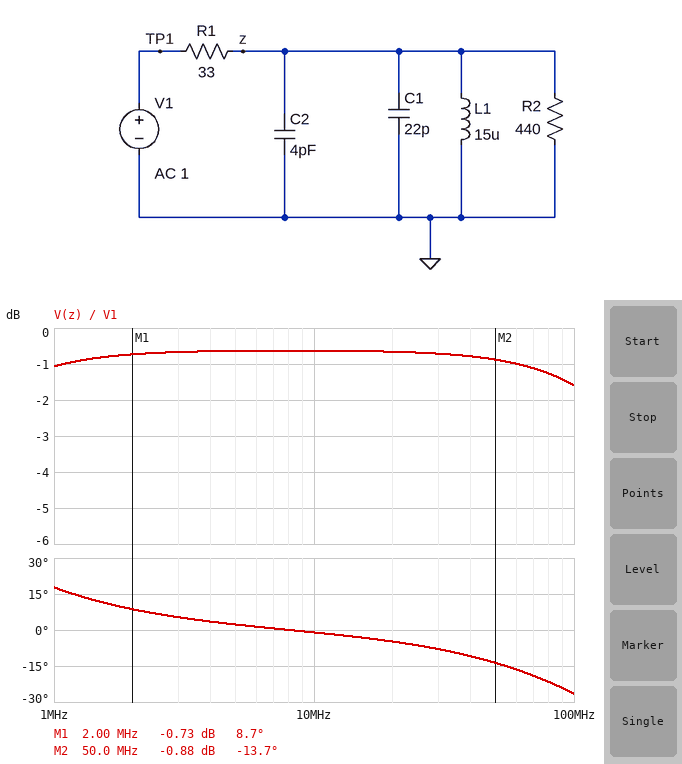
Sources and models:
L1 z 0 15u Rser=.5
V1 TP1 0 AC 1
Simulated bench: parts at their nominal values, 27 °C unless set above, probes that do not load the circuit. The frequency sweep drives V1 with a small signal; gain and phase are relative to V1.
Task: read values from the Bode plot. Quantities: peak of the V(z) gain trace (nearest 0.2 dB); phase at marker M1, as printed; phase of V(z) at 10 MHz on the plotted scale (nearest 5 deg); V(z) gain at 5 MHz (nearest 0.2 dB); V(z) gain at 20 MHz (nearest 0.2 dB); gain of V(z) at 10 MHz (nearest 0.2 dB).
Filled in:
-0.6 dB
8.7 deg
0 deg
-0.6 dB
-0.6 dB
-0.6 dB
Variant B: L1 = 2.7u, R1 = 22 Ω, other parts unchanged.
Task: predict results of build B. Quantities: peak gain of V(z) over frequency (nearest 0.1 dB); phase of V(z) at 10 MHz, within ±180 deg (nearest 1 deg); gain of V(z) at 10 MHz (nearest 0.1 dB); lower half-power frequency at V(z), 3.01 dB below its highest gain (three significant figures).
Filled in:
-0.4 dB
5 deg
-0.5 dB
1.26 MHz
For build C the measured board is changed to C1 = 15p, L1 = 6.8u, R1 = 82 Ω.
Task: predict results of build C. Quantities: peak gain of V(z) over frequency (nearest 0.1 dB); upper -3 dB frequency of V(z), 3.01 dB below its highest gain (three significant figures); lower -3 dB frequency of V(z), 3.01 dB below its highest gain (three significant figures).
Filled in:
-1.5 dB
123 MHz
1.61 MHz
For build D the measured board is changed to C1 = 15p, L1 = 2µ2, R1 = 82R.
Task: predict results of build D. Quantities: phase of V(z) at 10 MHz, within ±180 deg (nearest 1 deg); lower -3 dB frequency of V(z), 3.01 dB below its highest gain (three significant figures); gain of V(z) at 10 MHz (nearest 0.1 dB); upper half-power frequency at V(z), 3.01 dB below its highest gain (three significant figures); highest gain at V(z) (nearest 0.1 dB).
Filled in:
23 deg
4.84 MHz
-2.2 dB
126 MHz
-1.5 dB
